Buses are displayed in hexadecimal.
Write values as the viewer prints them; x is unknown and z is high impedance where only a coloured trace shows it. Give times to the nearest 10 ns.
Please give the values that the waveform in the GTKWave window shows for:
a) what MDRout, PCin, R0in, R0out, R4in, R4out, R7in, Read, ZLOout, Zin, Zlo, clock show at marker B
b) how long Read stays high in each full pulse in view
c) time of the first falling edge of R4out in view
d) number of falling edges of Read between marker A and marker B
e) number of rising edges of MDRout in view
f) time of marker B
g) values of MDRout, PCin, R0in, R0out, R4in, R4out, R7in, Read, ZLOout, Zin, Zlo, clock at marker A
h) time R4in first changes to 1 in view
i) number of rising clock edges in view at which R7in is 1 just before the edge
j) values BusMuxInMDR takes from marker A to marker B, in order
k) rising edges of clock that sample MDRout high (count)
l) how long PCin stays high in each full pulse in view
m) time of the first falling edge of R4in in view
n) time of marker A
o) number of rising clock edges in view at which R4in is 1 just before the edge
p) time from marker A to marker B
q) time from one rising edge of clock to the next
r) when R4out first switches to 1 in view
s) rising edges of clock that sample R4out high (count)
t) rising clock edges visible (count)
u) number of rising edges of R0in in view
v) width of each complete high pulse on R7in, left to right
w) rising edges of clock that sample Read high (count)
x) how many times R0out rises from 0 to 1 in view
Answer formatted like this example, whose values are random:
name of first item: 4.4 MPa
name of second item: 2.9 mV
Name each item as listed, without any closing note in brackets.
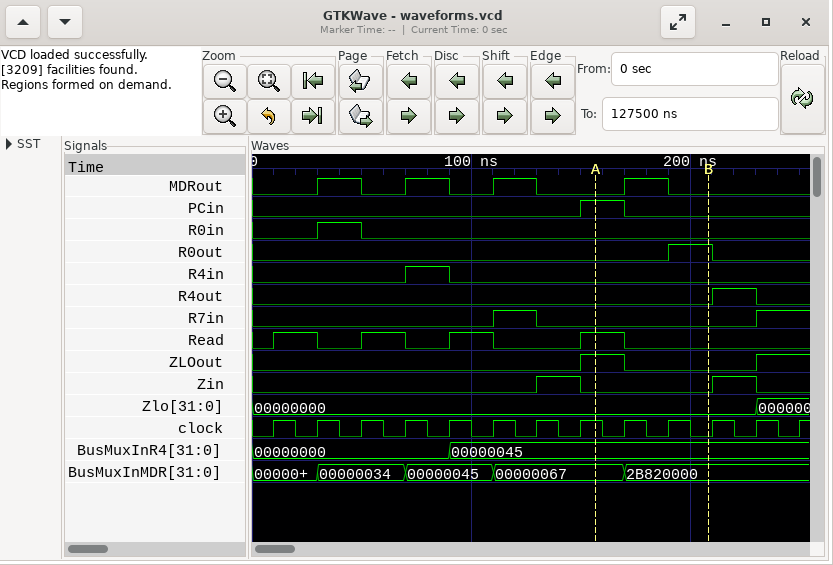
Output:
what MDRout, PCin, R0in, R0out, R4in, R4out, R7in, Read, ZLOout, Zin, Zlo, clock show at marker B: MDRout=0, PCin=0, R0in=0, R0out=1, R4in=0, R4out=0, R7in=0, Read=0, ZLOout=0, Zin=0, Zlo=00000000, clock=0
how long Read stays high in each full pulse in view: 20 ns, 20 ns, 20 ns, 20 ns
time of the first falling edge of R4out in view: 230 ns
number of falling edges of Read between marker A and marker B: 1
number of rising edges of MDRout in view: 4
time of marker B: 210 ns
values of MDRout, PCin, R0in, R0out, R4in, R4out, R7in, Read, ZLOout, Zin, Zlo, clock at marker A: MDRout=0, PCin=1, R0in=0, R0out=0, R4in=0, R4out=0, R7in=0, Read=1, ZLOout=1, Zin=0, Zlo=00000000, clock=1
time R4in first changes to 1 in view: 70 ns
number of rising clock edges in view at which R7in is 1 just before the edge: 2
values BusMuxInMDR takes from marker A to marker B, in order: 00000067, 2B820000
rising edges of clock that sample MDRout high: 4
how long PCin stays high in each full pulse in view: 20 ns
time of the first falling edge of R4in in view: 90 ns
time of marker A: 160 ns
number of rising clock edges in view at which R4in is 1 just before the edge: 1
time from marker A to marker B: 50 ns
time from one rising edge of clock to the next: 20 ns
when R4out first switches to 1 in view: 210 ns
rising edges of clock that sample R4out high: 1
rising clock edges visible: 13
number of rising edges of R0in in view: 1
width of each complete high pulse on R7in, left to right: 20 ns
rising edges of clock that sample Read high: 4
how many times R0out rises from 0 to 1 in view: 1
